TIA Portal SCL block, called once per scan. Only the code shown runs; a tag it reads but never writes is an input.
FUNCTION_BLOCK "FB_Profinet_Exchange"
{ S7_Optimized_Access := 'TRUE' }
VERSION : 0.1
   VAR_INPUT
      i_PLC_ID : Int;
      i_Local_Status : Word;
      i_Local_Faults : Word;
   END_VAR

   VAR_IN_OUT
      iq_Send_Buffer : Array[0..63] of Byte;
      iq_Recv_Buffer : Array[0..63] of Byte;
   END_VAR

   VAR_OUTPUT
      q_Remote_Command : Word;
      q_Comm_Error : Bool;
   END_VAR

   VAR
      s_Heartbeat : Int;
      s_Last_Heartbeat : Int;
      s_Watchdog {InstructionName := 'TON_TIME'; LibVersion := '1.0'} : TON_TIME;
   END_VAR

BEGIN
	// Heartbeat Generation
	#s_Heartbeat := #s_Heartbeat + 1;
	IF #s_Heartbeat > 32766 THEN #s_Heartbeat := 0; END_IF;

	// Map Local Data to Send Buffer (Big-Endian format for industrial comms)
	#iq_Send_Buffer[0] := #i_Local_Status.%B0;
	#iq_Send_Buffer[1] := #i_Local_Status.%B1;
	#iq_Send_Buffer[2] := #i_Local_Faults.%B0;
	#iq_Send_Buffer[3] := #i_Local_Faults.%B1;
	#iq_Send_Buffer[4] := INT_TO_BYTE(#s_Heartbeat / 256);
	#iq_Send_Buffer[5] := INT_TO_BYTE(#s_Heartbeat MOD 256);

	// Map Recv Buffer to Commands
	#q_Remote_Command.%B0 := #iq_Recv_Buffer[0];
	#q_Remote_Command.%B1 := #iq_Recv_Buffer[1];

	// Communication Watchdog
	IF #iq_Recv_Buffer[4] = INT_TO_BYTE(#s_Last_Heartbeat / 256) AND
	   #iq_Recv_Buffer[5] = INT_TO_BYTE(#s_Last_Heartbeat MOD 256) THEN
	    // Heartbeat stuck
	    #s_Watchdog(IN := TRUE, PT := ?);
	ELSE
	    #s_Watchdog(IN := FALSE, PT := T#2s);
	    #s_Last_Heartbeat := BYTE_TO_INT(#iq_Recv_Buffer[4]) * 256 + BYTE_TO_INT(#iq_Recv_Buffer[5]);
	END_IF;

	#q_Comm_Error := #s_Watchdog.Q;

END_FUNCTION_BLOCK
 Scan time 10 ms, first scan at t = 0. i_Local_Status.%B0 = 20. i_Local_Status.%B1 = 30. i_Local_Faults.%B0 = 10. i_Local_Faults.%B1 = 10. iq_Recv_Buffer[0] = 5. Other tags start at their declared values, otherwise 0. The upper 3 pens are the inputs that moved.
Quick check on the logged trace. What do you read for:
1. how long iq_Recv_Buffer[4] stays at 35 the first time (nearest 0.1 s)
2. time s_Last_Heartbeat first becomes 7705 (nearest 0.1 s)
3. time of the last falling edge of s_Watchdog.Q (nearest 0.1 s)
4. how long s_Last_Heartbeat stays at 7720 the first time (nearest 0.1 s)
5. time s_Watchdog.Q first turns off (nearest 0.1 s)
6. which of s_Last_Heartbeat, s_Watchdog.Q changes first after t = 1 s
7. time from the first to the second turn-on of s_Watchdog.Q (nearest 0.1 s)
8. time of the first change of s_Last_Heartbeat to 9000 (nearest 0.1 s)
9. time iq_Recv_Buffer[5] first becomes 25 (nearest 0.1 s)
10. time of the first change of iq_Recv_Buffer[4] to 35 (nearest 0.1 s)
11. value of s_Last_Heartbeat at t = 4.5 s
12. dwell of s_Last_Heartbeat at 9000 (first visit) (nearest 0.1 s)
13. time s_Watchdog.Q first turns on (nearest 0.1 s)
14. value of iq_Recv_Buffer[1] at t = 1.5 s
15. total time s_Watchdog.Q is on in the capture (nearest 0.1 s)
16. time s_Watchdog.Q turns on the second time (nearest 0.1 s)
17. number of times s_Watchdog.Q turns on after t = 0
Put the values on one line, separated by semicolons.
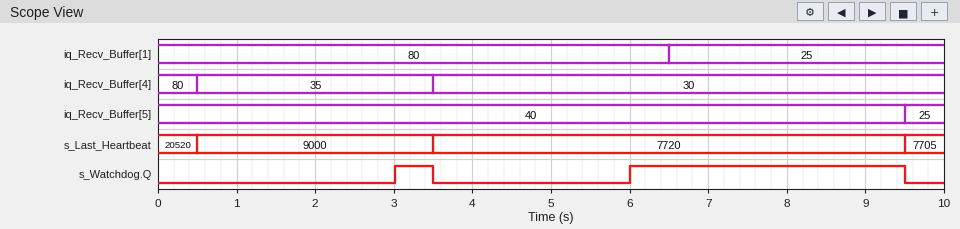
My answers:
3.0 s; 9.5 s; 9.5 s; 6.0 s; 3.5 s; s_Watchdog.Q; 3.0 s; 0.5 s; 9.5 s; 0.5 s; 7720; 3.0 s; 3.0 s; 80; 4.0 s; 6.0 s; 2
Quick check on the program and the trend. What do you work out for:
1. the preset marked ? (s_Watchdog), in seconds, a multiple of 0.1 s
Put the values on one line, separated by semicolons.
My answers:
2.5 s
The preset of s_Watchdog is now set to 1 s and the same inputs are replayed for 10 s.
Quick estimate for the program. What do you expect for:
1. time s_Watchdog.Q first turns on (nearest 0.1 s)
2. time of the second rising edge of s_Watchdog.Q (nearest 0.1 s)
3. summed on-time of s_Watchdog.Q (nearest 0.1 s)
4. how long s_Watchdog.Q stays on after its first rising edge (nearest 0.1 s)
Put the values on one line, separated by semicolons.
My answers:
1.5 s; 4.5 s; 7.0 s; 2.0 s
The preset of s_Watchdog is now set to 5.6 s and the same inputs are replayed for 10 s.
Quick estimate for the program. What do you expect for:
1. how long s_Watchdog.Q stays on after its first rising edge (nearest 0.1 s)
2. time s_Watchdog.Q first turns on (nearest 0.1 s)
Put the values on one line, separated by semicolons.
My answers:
0.4 s; 9.1 s
